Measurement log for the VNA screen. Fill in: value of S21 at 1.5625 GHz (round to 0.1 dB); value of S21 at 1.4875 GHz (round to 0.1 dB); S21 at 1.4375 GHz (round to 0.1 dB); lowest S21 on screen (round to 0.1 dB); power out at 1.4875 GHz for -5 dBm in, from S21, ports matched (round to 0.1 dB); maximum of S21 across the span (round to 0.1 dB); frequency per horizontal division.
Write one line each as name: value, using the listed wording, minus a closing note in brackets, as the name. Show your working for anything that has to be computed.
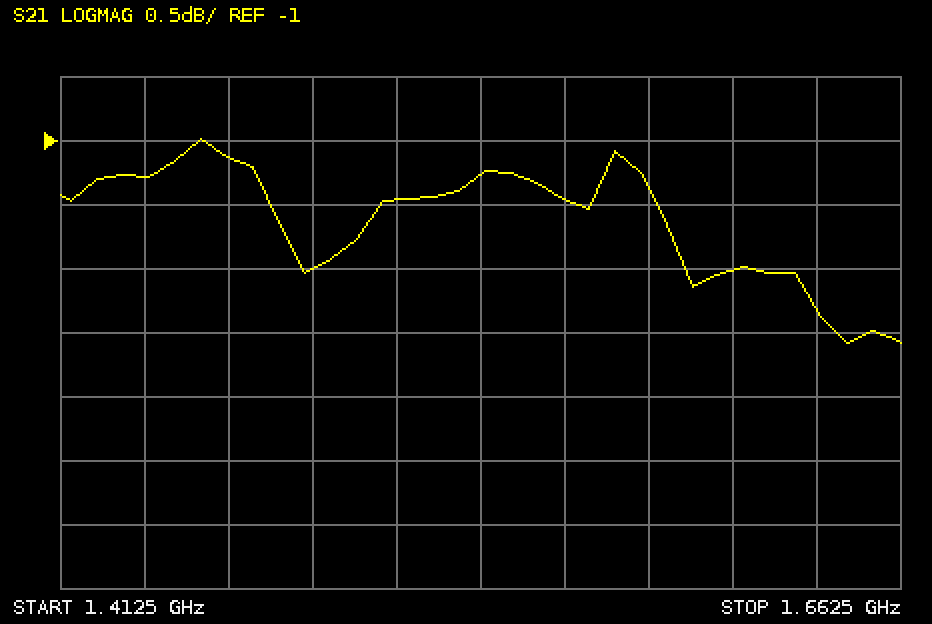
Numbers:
value of S21 at 1.5625 GHz: -1.5 dB
value of S21 at 1.4875 GHz: -2.0 dB
S21 at 1.4375 GHz: -1.3 dB
lowest S21 on screen: -2.6 dB
power out at 1.4875 GHz for -5 dBm in, from S21, ports matched: -5 dBm + (-2.0 dB) = -7.0 dBm
maximum of S21 across the span: -1.0 dB
frequency per horizontal division: 25 MHz
